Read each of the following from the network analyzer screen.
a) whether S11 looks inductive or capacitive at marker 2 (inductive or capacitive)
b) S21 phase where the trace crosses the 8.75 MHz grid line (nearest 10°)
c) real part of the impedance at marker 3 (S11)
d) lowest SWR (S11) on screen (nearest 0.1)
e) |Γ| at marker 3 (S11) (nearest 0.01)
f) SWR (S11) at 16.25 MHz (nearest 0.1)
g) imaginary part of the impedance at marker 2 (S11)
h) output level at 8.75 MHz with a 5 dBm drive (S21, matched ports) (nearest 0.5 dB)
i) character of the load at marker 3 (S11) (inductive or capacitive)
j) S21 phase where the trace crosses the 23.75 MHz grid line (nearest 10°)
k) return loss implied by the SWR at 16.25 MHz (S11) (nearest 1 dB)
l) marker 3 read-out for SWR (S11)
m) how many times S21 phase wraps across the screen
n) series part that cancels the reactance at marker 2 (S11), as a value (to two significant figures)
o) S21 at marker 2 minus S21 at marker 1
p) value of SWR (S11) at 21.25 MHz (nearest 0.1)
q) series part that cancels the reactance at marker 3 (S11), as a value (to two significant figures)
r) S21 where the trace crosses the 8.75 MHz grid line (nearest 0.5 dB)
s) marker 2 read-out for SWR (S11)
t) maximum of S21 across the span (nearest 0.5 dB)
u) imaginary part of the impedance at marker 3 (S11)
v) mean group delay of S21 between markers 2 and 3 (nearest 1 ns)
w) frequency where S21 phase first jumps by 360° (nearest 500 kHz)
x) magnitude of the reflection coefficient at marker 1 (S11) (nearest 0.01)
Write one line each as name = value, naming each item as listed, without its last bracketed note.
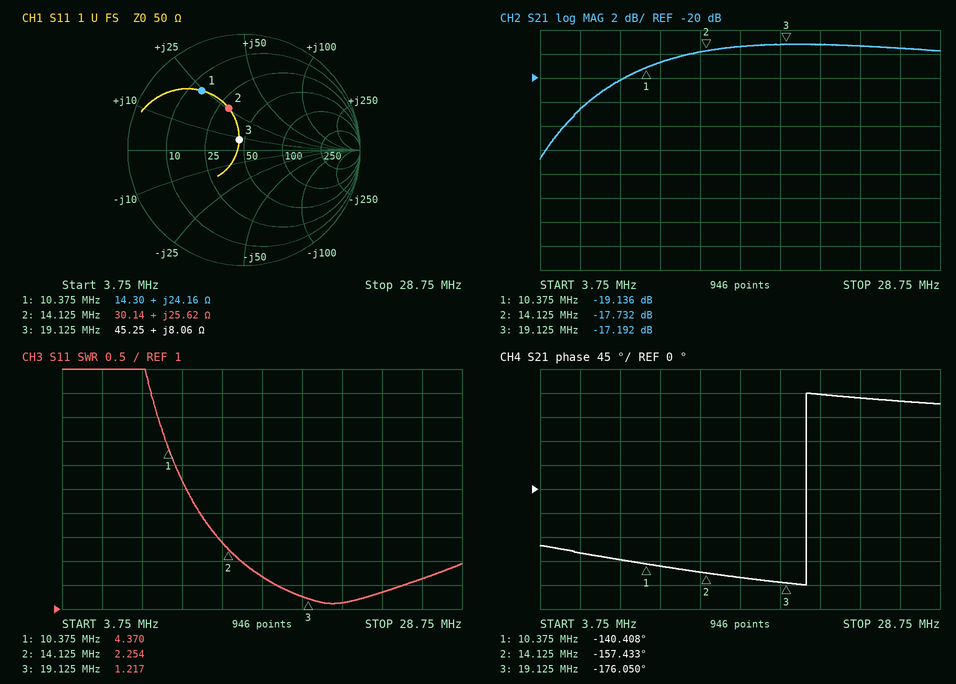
whether S11 looks inductive or capacitive at marker 2 = inductive
S21 phase where the trace crosses the 8.75 MHz grid line = -130°
real part of the impedance at marker 3 = 45.25 Ω
lowest SWR (S11) on screen = 1.1
|Γ| at marker 3 (S11) = 0.10
SWR (S11) at 16.25 MHz = 1.7
imaginary part of the impedance at marker 2 = +25.62 Ω
output level at 8.75 MHz with a 5 dBm drive (S21, matched ports) = -15.0 dBm
character of the load at marker 3 (S11) = inductive
S21 phase where the trace crosses the 23.75 MHz grid line = 170°
return loss implied by the SWR at 16.25 MHz (S11) = 12 dB
marker 3 read-out for SWR = 1.217
how many times S21 phase wraps across the screen = 1
series part that cancels the reactance at marker 2 (S11), as a value = 440 pF
S21 at marker 2 minus S21 at marker 1 = 1.404 dB
value of SWR (S11) at 21.25 MHz = 1.1
series part that cancels the reactance at marker 3 (S11), as a value = 1.0 nF
S21 where the trace crosses the 8.75 MHz grid line = -20.0 dB
marker 2 read-out for SWR = 2.254
maximum of S21 across the span = -17.0 dB
imaginary part of the impedance at marker 3 = +8.06 Ω
mean group delay of S21 between markers 2 and 3 = 10 ns
frequency where S21 phase first jumps by 360° = 20.5 MHz
magnitude of the reflection coefficient at marker 1 (S11) = 0.63
